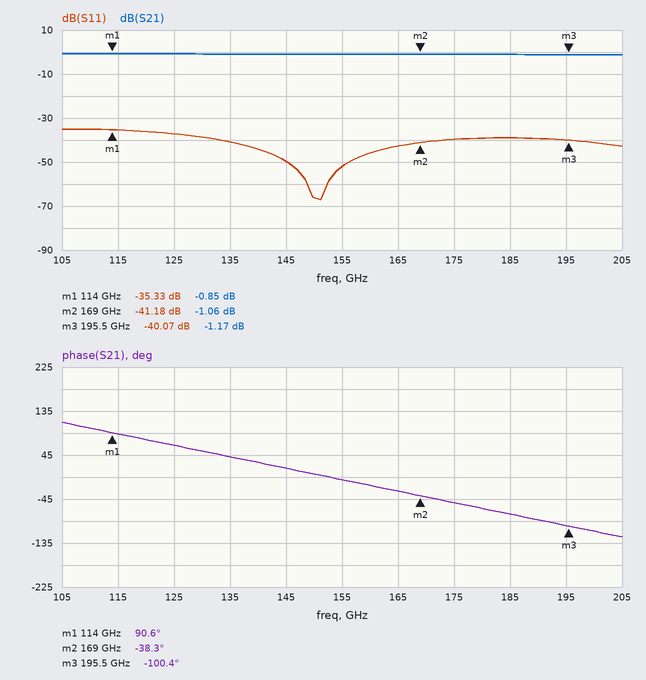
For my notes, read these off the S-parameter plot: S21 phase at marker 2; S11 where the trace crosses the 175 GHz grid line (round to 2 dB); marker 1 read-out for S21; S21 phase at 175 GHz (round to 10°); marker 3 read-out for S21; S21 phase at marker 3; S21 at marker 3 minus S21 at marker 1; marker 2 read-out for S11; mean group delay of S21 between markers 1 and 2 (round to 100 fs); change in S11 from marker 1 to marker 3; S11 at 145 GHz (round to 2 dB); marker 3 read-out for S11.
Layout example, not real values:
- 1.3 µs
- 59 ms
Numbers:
- -38.3°
- -40 dB
- -0.85 dB
- -50°
- -1.17 dB
- -100.4°
- -0.32 dB
- -41.18 dB
- 6.5 ps
- -4.74 dB
- -50 dB
- -40.07 dB
